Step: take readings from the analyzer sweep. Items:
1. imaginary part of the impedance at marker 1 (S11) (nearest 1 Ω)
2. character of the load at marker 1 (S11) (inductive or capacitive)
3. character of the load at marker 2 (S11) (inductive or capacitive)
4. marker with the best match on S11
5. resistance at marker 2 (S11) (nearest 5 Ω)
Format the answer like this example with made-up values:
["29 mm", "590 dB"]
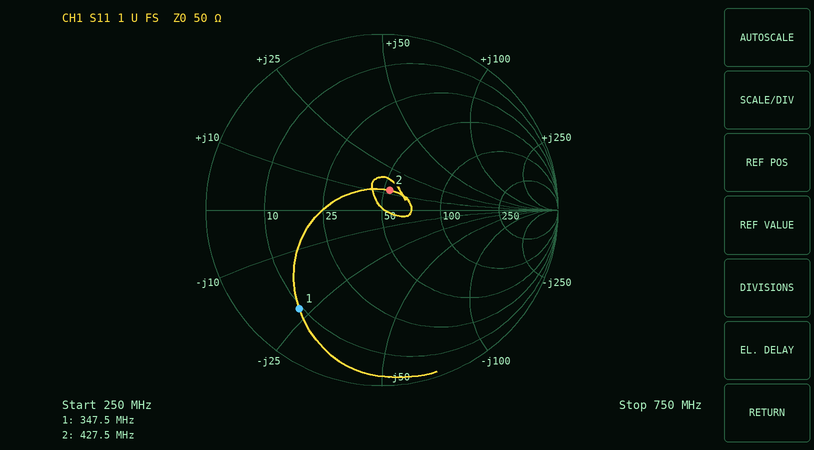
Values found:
["-23 Ω", "capacitive", "inductive", "marker 2", "55 Ω"]
